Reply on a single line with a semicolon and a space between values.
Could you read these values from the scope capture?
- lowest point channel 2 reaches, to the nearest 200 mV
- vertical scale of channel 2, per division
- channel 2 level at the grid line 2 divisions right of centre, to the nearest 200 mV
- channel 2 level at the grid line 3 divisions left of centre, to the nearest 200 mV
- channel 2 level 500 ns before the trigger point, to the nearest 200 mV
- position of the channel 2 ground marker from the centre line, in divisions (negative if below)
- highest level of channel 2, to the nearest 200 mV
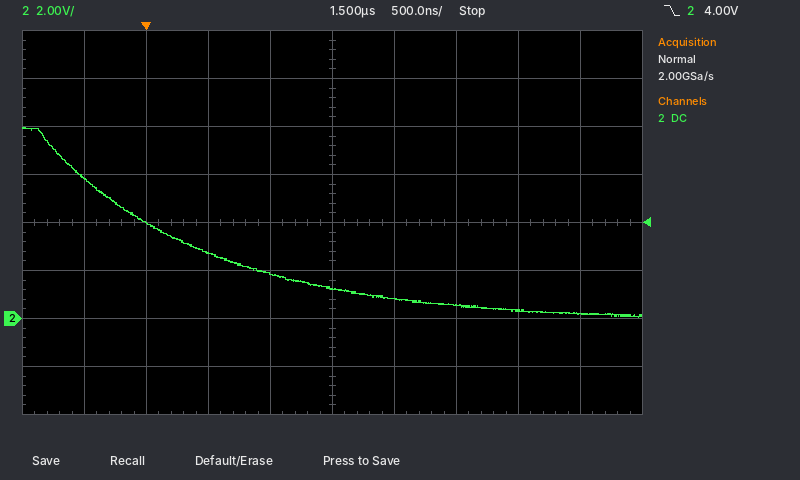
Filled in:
0.0 V; 2 V; 600 mV; 4.0 V; 5.8 V; -2.0 div; 8.0 V
